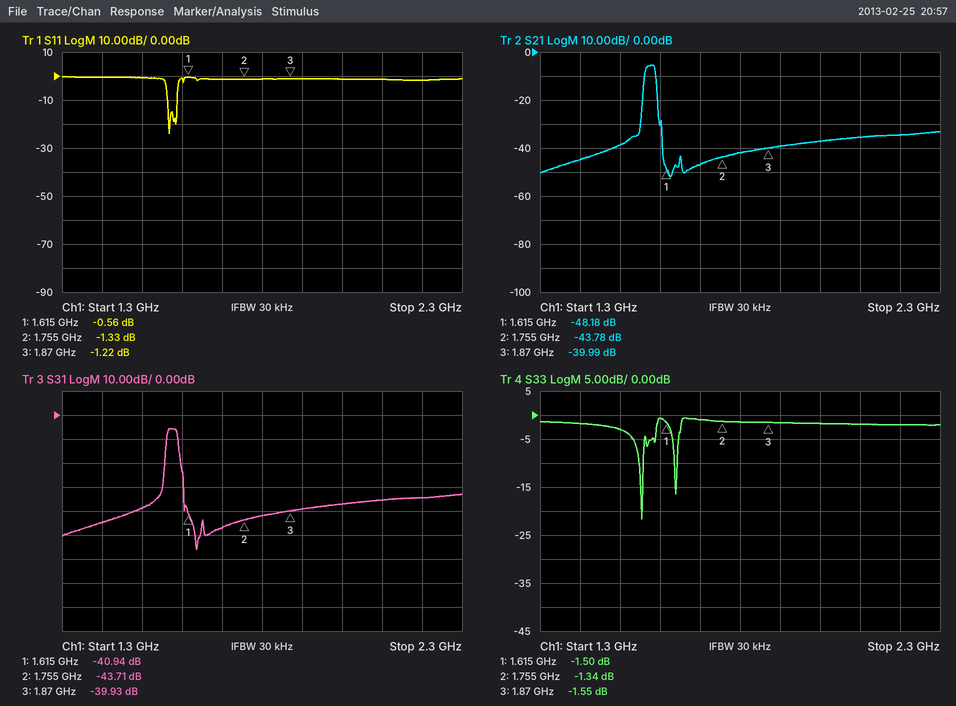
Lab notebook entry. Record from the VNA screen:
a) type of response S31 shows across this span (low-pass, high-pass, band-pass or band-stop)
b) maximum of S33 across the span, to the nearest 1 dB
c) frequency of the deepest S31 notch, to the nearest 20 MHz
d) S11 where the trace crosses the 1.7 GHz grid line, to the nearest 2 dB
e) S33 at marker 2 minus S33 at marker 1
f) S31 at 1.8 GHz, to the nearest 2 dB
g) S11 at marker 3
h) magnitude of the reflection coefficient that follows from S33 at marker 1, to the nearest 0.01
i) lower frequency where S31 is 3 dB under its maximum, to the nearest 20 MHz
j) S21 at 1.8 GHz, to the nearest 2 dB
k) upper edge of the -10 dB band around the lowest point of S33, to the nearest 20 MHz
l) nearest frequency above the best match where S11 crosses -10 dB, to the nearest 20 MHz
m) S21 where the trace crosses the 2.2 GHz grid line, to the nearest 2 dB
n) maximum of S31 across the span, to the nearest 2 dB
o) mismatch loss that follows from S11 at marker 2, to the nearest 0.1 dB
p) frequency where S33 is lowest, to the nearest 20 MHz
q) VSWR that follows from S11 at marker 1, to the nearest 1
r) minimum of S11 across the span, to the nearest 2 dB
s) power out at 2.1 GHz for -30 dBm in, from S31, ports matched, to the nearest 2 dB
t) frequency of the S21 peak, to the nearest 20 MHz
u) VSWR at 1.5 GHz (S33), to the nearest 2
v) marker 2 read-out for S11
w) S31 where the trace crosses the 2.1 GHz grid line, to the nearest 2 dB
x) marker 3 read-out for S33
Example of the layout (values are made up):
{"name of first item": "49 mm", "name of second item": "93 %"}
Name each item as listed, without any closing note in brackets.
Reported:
{"type of response S31 shows across this span": "band-pass", "maximum of S33 across the span, to the nearest 1 dB": "-1 dB", "frequency of the deepest S31 notch, to the nearest 20 MHz": "1.64 GHz", "S11 where the trace crosses the 1.7 GHz grid line, to the nearest 2 dB": "-2 dB", "S33 at marker 2 minus S33 at marker 1": "0.16 dB", "S31 at 1.8 GHz, to the nearest 2 dB": "-42 dB", "S11 at marker 3": "-1.22 dB", "magnitude of the reflection coefficient that follows from S33 at marker 1, to the nearest 0.01": "0.84", "lower frequency where S31 is 3 dB under its maximum, to the nearest 20 MHz": "1.56 GHz", "S21 at 1.8 GHz, to the nearest 2 dB": "-42 dB", "upper edge of the -10 dB band around the lowest point of S33, to the nearest 20 MHz": "1.56 GHz", "nearest frequency above the best match where S11 crosses -10 dB, to the nearest 20 MHz": "1.58 GHz", "S21 where the trace crosses the 2.2 GHz grid line, to the nearest 2 dB": "-34 dB", "maximum of S31 across the span, to the nearest 2 dB": "-6 dB", "mismatch loss that follows from S11 at marker 2, to the nearest 0.1 dB": "5.8 dB", "frequency where S33 is lowest, to the nearest 20 MHz": "1.56 GHz", "VSWR that follows from S11 at marker 1, to the nearest 1": "31", "minimum of S11 across the span, to the nearest 2 dB": "-24 dB", "power out at 2.1 GHz for -30 dBm in, from S31, ports matched, to the nearest 2 dB": "-66 dBm", "frequency of the S21 peak, to the nearest 20 MHz": "1.58 GHz", "VSWR at 1.5 GHz (S33), to the nearest 2": "6", "marker 2 read-out for S11": "-1.33 dB", "S31 where the trace crosses the 2.1 GHz grid line, to the nearest 2 dB": "-36 dB", "marker 3 read-out for S33": "-1.55 dB"}
